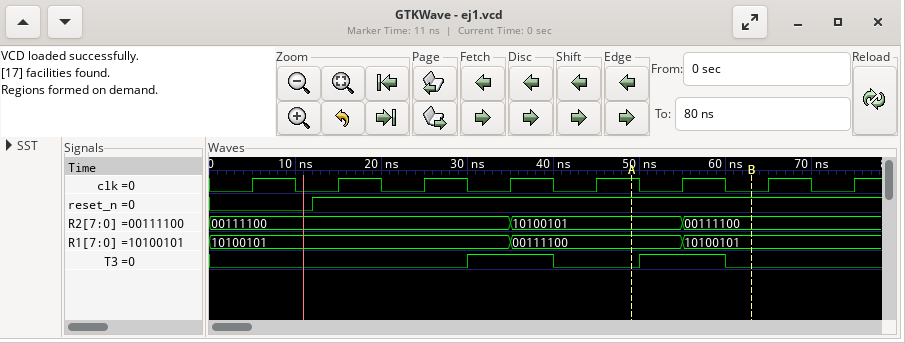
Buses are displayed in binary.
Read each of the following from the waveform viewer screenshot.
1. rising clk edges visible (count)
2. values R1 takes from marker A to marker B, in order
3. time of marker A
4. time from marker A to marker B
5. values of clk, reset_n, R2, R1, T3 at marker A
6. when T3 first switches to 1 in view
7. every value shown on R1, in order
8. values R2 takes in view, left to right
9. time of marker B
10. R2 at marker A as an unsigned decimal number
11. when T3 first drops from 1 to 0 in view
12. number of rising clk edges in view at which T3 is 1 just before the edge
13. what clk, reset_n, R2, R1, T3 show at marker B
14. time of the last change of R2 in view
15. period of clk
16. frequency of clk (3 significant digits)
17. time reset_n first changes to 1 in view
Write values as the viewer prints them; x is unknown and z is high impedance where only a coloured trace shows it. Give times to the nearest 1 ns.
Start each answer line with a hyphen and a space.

- 8
- 00111100, 10100101
- 49 ns
- 14 ns
- clk=1, reset_n=1, R2=10100101, R1=00111100, T3=0
- 30 ns
- 10100101, 00111100, 10100101
- 00111100, 10100101, 00111100
- 63 ns
- 165
- 40 ns
- 2
- clk=0, reset_n=1, R2=00111100, R1=10100101, T3=0
- 55 ns
- 10 ns
- 100 MHz
- 12 ns
